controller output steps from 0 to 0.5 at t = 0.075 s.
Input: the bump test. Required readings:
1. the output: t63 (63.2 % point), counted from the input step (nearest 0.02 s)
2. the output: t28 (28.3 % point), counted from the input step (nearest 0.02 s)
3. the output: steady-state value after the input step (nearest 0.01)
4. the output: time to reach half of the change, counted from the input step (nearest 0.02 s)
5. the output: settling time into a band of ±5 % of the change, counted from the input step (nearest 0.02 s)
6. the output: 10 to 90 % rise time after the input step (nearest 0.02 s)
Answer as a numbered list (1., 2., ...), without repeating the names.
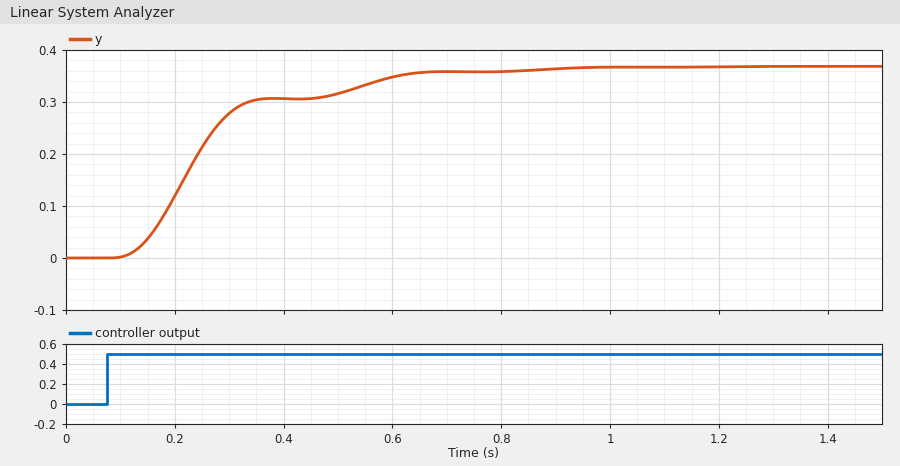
1. 0.18 s
2. 0.12 s
3. 0.37
4. 0.16 s
5. 0.54 s
6. 0.40 s
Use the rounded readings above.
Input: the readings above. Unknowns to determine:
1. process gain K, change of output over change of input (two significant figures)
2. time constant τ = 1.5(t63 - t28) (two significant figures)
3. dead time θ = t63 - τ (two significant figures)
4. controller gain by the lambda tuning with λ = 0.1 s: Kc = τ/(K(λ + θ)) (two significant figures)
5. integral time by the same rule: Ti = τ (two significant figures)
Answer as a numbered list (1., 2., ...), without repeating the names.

1. 0.74
2. 0.090 s
3. 0.090 s
4. 0.64
5. 0.090 s
